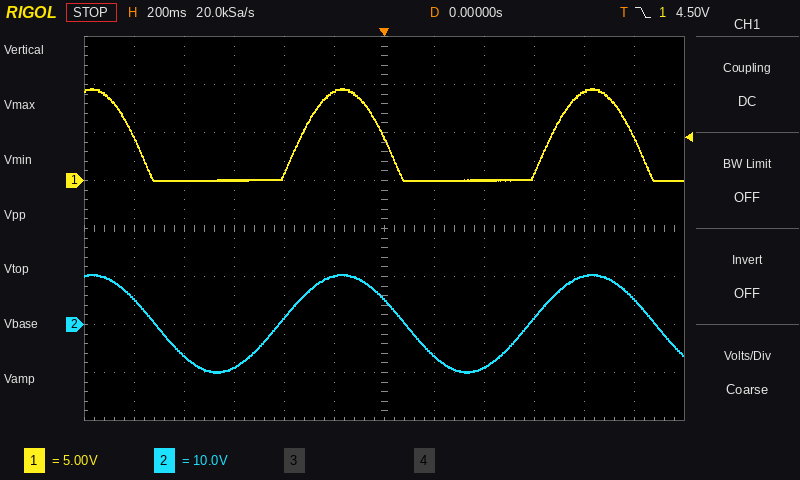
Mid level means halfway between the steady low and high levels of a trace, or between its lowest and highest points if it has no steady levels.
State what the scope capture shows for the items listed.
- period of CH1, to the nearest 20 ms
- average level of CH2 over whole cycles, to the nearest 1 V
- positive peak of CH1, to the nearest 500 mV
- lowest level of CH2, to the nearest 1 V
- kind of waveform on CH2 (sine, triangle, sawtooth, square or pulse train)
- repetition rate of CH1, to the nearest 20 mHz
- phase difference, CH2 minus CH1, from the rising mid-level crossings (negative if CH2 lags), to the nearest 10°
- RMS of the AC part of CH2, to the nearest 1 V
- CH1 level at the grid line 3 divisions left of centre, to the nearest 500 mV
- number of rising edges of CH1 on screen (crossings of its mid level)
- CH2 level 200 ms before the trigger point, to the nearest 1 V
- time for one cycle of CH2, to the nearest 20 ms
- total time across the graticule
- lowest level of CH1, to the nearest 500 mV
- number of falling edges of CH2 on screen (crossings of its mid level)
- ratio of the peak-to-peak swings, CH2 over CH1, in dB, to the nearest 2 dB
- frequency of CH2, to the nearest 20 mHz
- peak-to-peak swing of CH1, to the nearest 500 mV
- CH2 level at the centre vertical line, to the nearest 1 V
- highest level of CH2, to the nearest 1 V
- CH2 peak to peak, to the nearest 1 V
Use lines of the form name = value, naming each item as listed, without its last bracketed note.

period of CH1, to the nearest 20 ms = 1.00 s
average level of CH2 over whole cycles, to the nearest 1 V = 0 V
positive peak of CH1, to the nearest 500 mV = 9.5 V
lowest level of CH2, to the nearest 1 V = -10 V
kind of waveform on CH2 = sine
repetition rate of CH1, to the nearest 20 mHz = 1.00 Hz
phase difference, CH2 minus CH1, from the rising mid-level crossings (negative if CH2 lags), to the nearest 10° = +30°
RMS of the AC part of CH2, to the nearest 1 V = 7 V
CH1 level at the grid line 3 divisions left of centre, to the nearest 500 mV = 0.0 V
number of rising edges of CH1 on screen = 2
CH2 level 200 ms before the trigger point, to the nearest 1 V = 10 V
time for one cycle of CH2, to the nearest 20 ms = 1.00 s
total time across the graticule = 2.4 s
lowest level of CH1, to the nearest 500 mV = 0.0 V
number of falling edges of CH2 on screen = 3
ratio of the peak-to-peak swings, CH2 over CH1, in dB, to the nearest 2 dB = 6 dB
frequency of CH2, to the nearest 20 mHz = 1.00 Hz
peak-to-peak swing of CH1, to the nearest 500 mV = 9.5 V
CH2 level at the centre vertical line, to the nearest 1 V = 5 V
highest level of CH2, to the nearest 1 V = 10 V
CH2 peak to peak, to the nearest 1 V = 20 V
